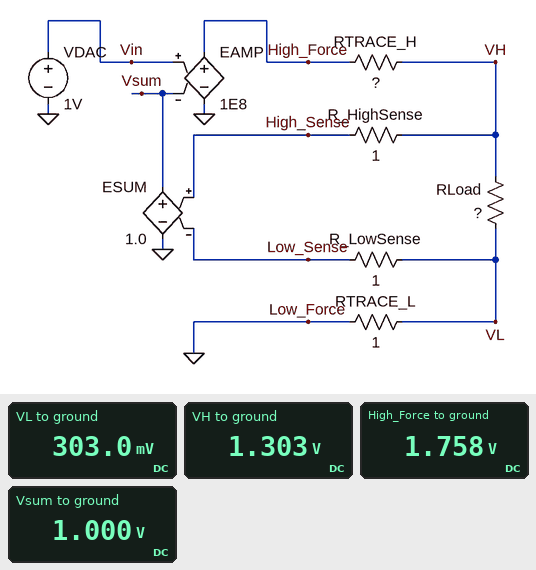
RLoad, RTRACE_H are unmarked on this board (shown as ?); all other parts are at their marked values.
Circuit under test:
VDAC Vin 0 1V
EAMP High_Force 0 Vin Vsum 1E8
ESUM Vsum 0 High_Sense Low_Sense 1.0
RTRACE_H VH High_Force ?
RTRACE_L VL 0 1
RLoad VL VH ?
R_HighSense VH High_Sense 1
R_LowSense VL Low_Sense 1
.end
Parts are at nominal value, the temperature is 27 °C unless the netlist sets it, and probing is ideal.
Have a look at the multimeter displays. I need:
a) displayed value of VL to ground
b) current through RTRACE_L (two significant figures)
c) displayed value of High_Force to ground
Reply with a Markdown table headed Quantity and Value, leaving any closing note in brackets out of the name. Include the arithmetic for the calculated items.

| Quantity | Value |
|---|---|
| displayed value of VL to ground | 303.0 mV |
| current through RTRACE_L | (303 mV) / 1 Ω = 300 mA |
| displayed value of High_Force to ground | 1.758 V |
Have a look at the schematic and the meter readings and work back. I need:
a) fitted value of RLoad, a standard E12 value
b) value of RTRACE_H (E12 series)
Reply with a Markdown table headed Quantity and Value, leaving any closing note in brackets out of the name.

| Quantity | Value |
|---|---|
| fitted value of RLoad, a standard E12 value | 3.3 Ω |
| value of RTRACE_H | 1.5 Ω |
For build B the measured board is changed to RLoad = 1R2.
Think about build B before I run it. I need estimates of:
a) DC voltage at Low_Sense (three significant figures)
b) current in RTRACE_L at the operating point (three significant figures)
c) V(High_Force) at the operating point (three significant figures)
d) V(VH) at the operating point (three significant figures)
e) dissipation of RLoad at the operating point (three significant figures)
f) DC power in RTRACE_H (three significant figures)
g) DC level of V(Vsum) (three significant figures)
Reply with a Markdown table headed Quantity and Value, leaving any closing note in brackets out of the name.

| Quantity | Value |
|---|---|
| DC voltage at Low_Sense | 833 mV |
| current in RTRACE_L at the operating point | 833 mA |
| V(High_Force) at the operating point | 3.08 V |
| V(VH) at the operating point | 1.83 V |
| dissipation of RLoad at the operating point | 833 mW |
| DC power in RTRACE_H | 1.04 W |
| DC level of V(Vsum) | 1.00 V |
